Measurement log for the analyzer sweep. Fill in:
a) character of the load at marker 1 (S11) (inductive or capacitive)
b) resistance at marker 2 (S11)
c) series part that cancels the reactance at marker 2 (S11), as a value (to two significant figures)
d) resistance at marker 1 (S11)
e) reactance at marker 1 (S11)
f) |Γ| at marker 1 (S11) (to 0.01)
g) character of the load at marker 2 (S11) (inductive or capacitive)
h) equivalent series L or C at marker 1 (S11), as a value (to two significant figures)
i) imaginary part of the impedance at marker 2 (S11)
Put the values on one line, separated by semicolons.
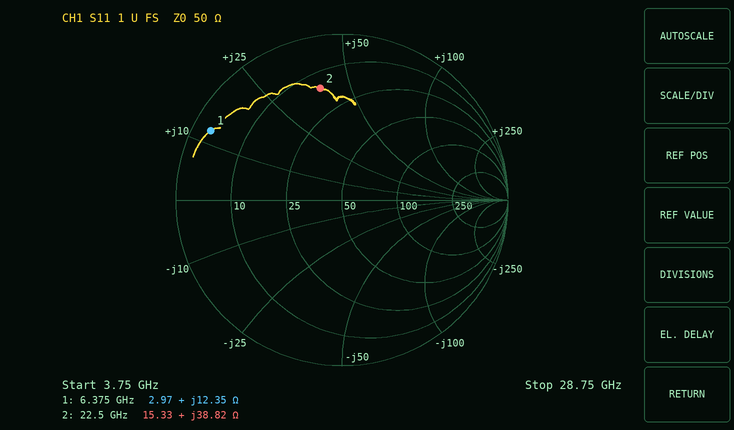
inductive; 15.33 Ω; 180 fF; 2.97 Ω; +12.35 Ω; 0.89; inductive; 310 pH; +38.82 Ω
